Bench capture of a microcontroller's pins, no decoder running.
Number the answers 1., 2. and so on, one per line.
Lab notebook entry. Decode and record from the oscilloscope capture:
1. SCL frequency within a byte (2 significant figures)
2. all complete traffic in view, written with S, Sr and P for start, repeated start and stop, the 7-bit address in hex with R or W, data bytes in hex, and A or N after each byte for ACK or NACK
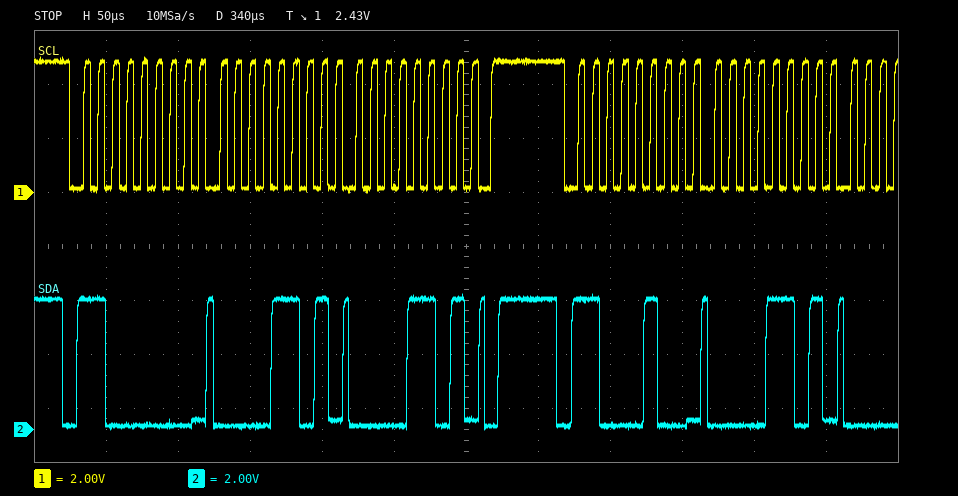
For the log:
1. 100 kHz
2. S 60W A 0D A 0D A P S 62W A 0D A
